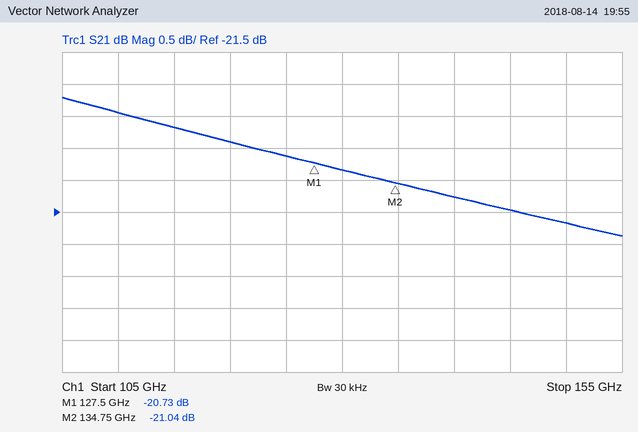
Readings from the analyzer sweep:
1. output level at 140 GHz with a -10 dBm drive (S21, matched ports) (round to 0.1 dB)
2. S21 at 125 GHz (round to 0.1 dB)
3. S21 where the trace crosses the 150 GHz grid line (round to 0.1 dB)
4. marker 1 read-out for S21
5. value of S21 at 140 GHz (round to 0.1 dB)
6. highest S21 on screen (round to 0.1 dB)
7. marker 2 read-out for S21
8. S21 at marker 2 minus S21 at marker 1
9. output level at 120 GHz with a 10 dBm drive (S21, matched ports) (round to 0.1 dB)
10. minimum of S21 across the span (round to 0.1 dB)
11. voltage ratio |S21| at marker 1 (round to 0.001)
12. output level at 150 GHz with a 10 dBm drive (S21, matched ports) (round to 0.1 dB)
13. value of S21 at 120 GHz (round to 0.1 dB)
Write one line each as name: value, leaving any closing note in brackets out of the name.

output level at 140 GHz with a -10 dBm drive (S21, matched ports): -31.3 dBm
S21 at 125 GHz: -20.6 dB
S21 where the trace crosses the 150 GHz grid line: -21.7 dB
marker 1 read-out for S21: -20.73 dB
value of S21 at 140 GHz: -21.3 dB
highest S21 on screen: -19.7 dB
marker 2 read-out for S21: -21.04 dB
S21 at marker 2 minus S21 at marker 1: -0.31 dB
output level at 120 GHz with a 10 dBm drive (S21, matched ports): -10.4 dBm
minimum of S21 across the span: -21.9 dB
voltage ratio |S21| at marker 1: 0.092
output level at 150 GHz with a 10 dBm drive (S21, matched ports): -11.7 dBm
value of S21 at 120 GHz: -20.4 dB
